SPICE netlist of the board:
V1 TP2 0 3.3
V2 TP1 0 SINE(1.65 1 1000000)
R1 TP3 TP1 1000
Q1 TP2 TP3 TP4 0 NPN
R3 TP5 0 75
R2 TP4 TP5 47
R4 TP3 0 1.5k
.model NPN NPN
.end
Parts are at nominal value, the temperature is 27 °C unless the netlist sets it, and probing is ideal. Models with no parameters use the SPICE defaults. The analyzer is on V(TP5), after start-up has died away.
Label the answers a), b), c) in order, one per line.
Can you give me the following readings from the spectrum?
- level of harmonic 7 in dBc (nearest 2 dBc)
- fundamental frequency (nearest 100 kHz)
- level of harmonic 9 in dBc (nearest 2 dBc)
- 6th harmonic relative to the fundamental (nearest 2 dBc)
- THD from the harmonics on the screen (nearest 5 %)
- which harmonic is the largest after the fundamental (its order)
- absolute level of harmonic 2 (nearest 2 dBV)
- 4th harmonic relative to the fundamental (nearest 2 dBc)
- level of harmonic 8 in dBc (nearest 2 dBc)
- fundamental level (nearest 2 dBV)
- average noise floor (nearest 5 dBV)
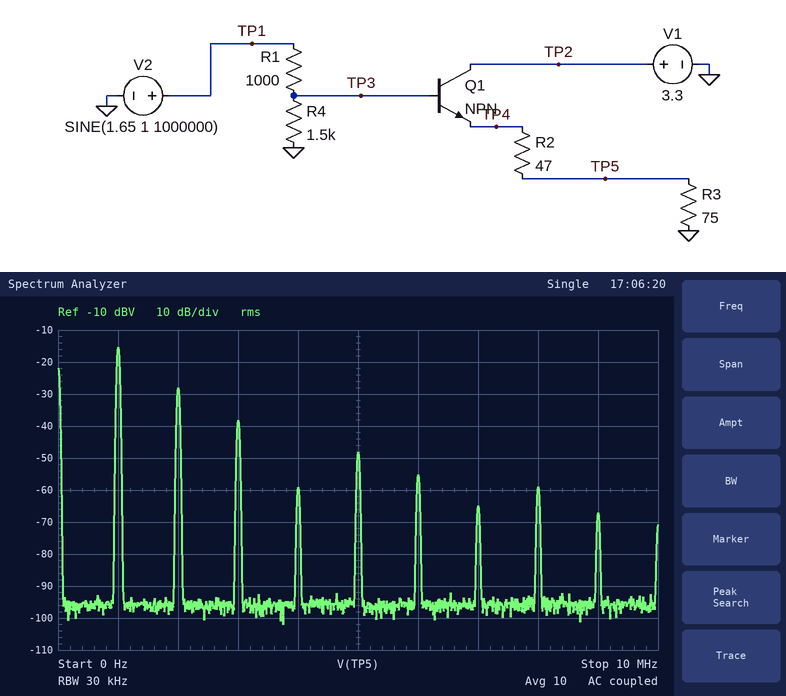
a) -50 dBc
b) 1.0 MHz
c) -52 dBc
d) -40 dBc
e) 25 %
f) 2
g) -28 dBV
h) -44 dBc
i) -44 dBc
j) -16 dBV
k) -95 dBV
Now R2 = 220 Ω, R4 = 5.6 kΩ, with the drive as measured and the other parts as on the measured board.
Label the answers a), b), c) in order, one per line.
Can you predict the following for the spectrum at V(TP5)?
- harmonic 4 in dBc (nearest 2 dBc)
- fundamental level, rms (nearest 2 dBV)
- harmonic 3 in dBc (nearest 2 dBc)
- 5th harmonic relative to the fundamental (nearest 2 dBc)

a) -32 dBc
b) -18 dBV
c) -28 dBc
d) -40 dBc
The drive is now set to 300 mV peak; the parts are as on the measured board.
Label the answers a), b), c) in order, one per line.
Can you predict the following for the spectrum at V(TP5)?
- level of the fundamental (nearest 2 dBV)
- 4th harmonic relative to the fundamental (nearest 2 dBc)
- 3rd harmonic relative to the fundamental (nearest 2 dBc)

a) -24 dBV
b) -56 dBc
c) -44 dBc
